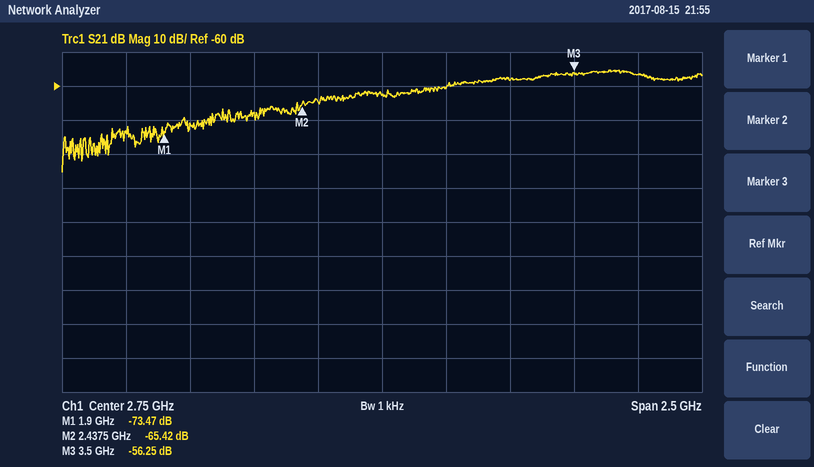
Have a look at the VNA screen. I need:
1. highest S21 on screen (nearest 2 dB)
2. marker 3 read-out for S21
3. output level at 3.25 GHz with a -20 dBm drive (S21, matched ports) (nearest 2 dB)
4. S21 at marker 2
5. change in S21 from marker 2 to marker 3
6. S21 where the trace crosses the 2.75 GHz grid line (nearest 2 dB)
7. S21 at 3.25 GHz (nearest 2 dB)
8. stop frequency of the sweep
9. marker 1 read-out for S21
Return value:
-56 dB
-56.25 dB
-78 dBm
-65.42 dB
9.17 dB
-62 dB
-58 dB
4 GHz
-73.47 dB
